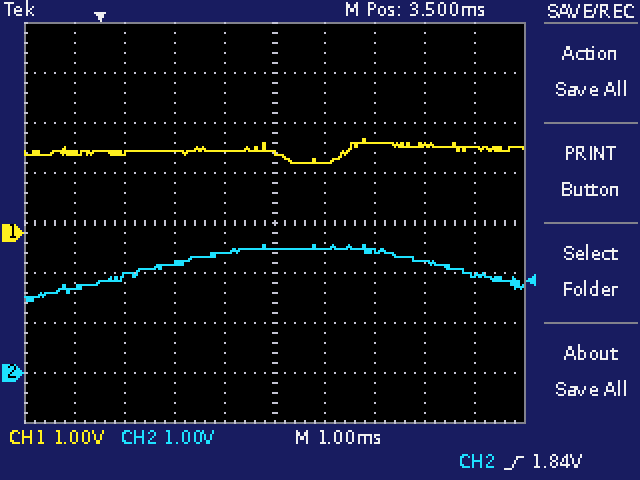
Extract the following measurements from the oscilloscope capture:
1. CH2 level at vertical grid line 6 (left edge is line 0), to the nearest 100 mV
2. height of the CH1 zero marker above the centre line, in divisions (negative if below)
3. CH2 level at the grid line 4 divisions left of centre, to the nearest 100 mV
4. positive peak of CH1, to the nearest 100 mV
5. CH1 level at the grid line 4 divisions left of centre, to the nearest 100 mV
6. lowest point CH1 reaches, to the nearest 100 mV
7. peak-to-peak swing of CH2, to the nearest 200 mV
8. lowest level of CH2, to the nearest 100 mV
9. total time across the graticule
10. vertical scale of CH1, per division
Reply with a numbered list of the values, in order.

1. 2.5 V
2. -0.2 div
3. 1.7 V
4. 1.9 V
5. 1.6 V
6. 1.4 V
7. 1.2 V
8. 1.4 V
9. 10 ms
10. 1 V
